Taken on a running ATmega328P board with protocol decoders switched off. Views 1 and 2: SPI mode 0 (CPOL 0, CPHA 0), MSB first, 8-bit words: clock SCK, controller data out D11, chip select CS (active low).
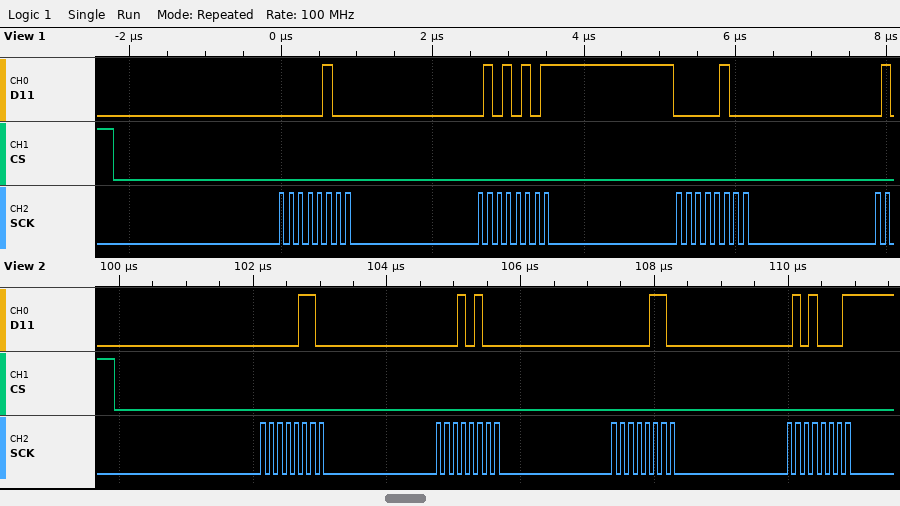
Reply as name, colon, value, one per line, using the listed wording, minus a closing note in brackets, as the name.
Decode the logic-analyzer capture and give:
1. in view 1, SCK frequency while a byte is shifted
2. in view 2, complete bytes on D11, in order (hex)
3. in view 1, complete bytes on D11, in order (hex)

in view 1, SCK frequency while a byte is shifted: 8 MHz
in view 2, complete bytes on D11, in order: 06 14 06 51
in view 1, complete bytes on D11, in order: 0x04 0x55 0x04
